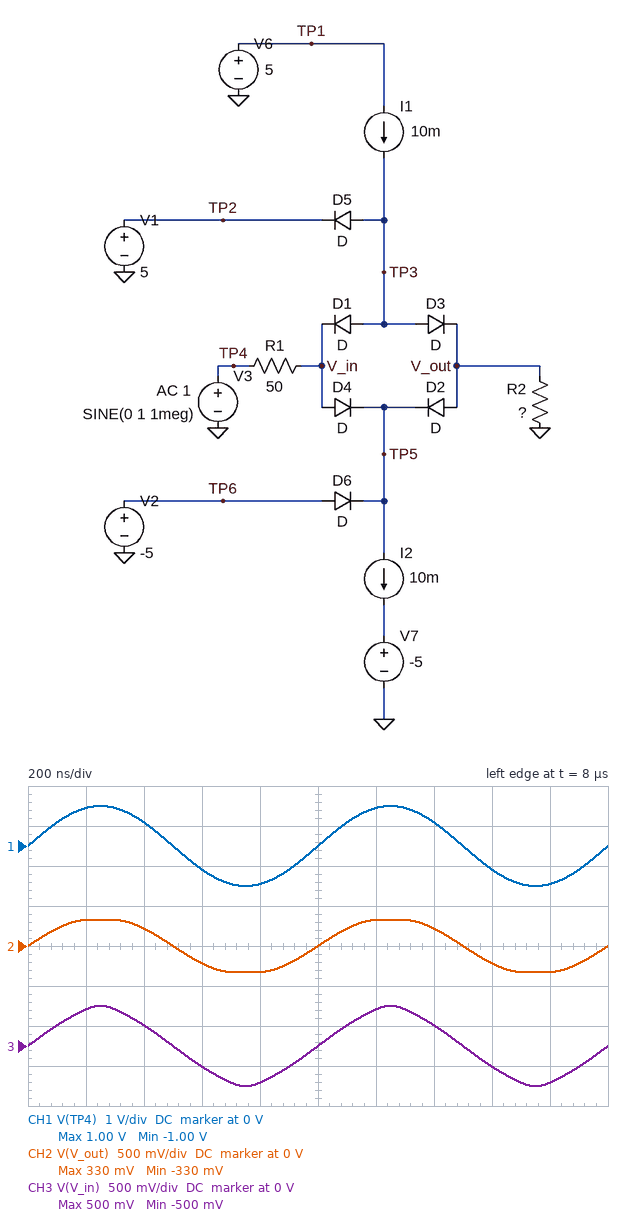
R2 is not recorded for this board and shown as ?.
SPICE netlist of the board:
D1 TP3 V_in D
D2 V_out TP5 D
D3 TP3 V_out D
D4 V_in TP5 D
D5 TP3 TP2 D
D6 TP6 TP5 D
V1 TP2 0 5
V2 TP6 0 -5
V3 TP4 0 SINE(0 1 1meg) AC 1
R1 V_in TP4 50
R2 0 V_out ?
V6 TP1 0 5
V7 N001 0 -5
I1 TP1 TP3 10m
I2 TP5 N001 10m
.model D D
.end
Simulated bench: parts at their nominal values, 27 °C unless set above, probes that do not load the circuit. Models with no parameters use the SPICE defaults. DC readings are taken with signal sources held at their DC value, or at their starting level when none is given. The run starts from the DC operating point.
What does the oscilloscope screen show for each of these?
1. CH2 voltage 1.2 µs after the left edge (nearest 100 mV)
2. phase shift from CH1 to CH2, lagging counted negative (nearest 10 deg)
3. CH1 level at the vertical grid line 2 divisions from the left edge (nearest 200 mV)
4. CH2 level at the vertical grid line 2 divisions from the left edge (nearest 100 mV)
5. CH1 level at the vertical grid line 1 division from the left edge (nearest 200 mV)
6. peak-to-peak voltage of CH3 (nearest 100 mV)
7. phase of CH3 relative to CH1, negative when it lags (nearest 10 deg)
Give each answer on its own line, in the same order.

300 mV
0 deg
600 mV
200 mV
1.0 V
1.0 V
0 deg
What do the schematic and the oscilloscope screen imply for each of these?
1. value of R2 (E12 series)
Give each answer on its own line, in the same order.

33 Ω
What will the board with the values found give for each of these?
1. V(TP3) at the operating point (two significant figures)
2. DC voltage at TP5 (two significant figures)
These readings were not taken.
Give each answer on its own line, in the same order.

700 mV
-700 mV
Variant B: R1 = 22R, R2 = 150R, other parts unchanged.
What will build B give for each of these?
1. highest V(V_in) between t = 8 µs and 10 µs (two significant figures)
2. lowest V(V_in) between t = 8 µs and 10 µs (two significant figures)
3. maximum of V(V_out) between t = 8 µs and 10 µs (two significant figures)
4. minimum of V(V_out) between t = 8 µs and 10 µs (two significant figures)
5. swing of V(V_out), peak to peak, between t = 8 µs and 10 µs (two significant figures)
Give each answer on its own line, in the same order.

880 mV
-880 mV
840 mV
-840 mV
1.7 V
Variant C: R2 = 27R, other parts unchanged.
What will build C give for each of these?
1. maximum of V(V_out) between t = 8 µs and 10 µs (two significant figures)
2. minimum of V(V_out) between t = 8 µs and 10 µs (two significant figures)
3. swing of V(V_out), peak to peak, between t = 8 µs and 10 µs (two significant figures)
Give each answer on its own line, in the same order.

270 mV
-270 mV
540 mV
